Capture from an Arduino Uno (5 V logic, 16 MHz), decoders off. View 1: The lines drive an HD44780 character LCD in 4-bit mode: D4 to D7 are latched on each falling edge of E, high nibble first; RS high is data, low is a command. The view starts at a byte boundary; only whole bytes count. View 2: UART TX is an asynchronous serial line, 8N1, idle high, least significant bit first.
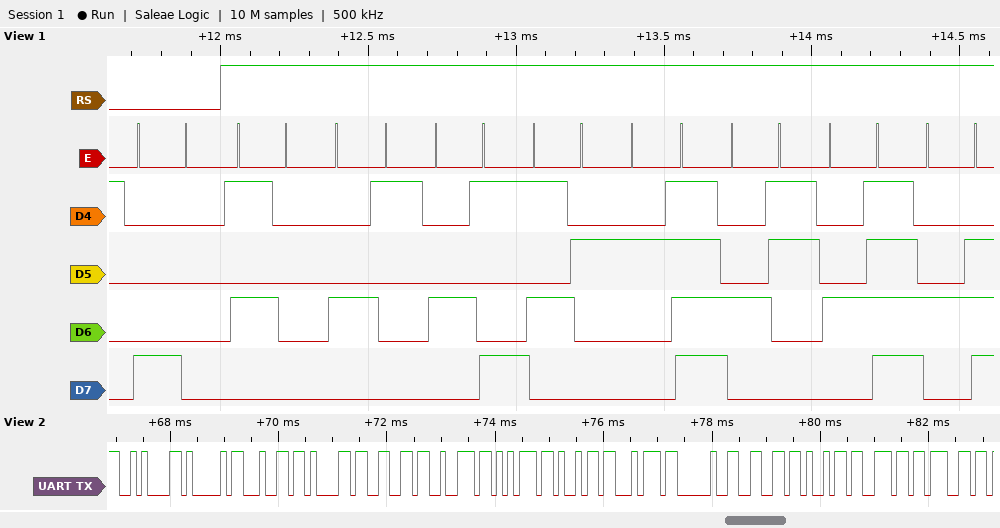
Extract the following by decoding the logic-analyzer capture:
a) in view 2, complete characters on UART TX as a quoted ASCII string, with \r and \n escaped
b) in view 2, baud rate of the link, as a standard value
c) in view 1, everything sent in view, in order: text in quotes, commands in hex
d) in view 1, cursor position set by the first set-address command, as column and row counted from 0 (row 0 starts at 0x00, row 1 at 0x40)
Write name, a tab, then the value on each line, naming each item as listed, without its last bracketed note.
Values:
in view 2, complete characters on UART TX as a quoted ASCII string, with \r and \n escaped	"\nAdafruit fing"
in view 2, baud rate of the link, as a standard value	9600 baud
in view 1, everything sent in view, in order: text in quotes, commands in hex	0x80 "PAIR/CON"
in view 1, cursor position set by the first set-address command, as column and row counted from 0	column 0, row 0
